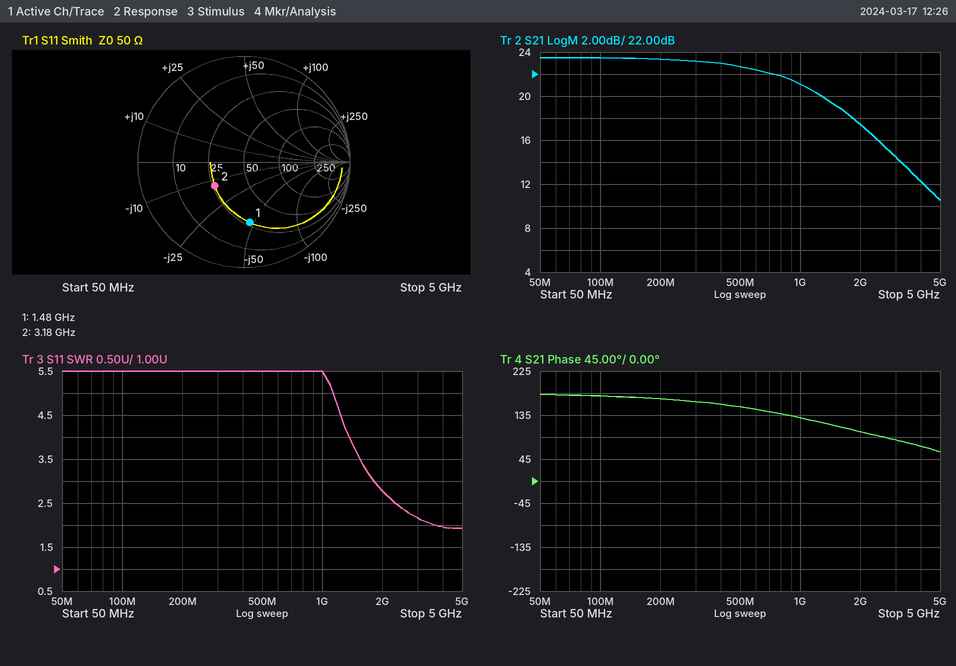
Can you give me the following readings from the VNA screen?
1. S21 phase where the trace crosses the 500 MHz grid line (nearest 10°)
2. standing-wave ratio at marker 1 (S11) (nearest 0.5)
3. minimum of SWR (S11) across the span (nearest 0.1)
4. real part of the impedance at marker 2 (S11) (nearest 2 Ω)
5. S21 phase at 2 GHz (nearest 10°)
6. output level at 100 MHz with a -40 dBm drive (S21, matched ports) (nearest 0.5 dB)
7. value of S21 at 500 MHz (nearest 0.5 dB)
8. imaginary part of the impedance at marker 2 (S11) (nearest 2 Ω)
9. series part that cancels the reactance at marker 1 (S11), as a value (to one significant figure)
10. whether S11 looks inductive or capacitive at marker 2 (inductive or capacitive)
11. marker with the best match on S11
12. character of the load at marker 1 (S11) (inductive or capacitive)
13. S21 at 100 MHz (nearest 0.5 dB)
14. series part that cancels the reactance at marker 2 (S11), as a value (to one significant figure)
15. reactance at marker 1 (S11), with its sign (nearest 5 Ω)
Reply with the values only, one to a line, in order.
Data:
150°
3.5
1.9
26 Ω
100°
-16.5 dBm
22.5 dB
-14 Ω
5 nH
capacitive
marker 2
capacitive
23.5 dB
700 pH
-45 Ω
